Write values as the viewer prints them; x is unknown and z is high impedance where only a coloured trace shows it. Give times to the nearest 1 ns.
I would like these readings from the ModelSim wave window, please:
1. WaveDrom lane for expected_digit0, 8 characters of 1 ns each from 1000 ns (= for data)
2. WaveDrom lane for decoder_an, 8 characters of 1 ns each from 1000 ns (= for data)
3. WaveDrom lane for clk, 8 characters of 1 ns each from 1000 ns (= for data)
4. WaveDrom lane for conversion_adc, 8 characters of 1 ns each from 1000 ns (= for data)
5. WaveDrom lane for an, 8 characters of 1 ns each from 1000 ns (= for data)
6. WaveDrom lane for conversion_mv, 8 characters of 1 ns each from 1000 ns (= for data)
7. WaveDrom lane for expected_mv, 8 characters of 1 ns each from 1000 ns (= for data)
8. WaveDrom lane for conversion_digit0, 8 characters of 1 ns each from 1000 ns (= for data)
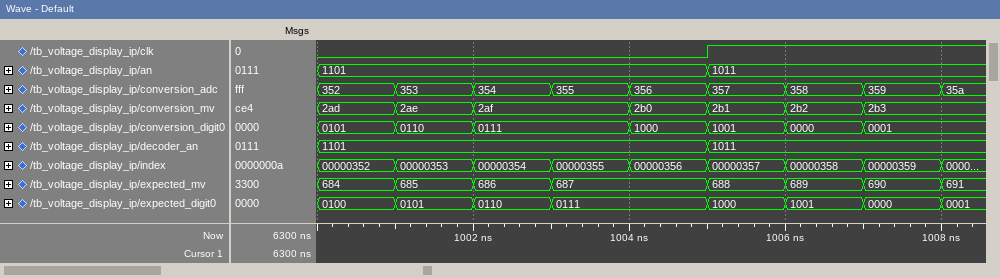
{name: 'expected_digit0', wave: '====.===', data: '0100 0101 0110 0111 1000 1001 0000'}
{name: 'decoder_an', wave: '=....=..', data: '1101 1011'}
{name: 'clk', wave: '0....1..'}
{name: 'conversion_adc', wave: '========', data: '352 353 354 355 356 357 358 359'}
{name: 'an', wave: '=....=..', data: '1101 1011'}
{name: 'conversion_mv', wave: '===.====', data: '2ad 2ae 2af 2b0 2b1 2b2 2b3'}
{name: 'expected_mv', wave: '====.===', data: '684 685 686 687 688 689 690'}
{name: 'conversion_digit0', wave: '===.====', data: '0101 0110 0111 1000 1001 0000 0001'}
